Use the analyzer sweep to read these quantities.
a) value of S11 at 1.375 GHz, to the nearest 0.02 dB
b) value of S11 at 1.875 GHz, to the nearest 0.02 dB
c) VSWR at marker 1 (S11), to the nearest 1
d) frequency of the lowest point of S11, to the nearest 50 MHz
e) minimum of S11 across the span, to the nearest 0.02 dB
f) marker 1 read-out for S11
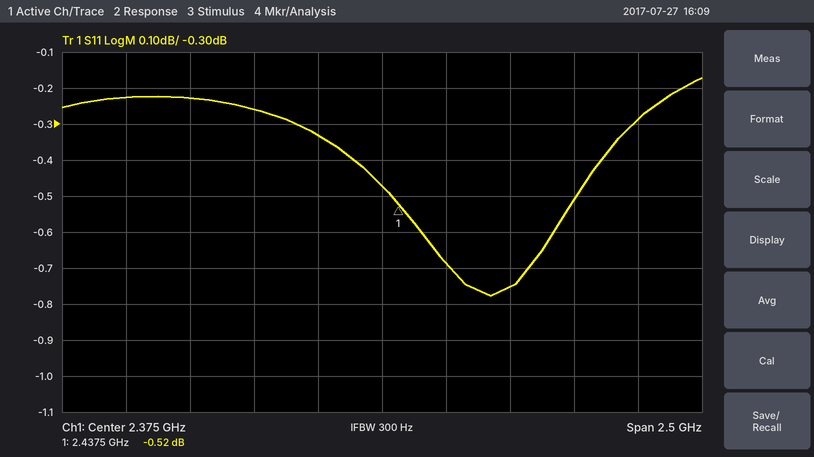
-0.22 dB
-0.26 dB
33
2.80 GHz
-0.78 dB
-0.52 dB
